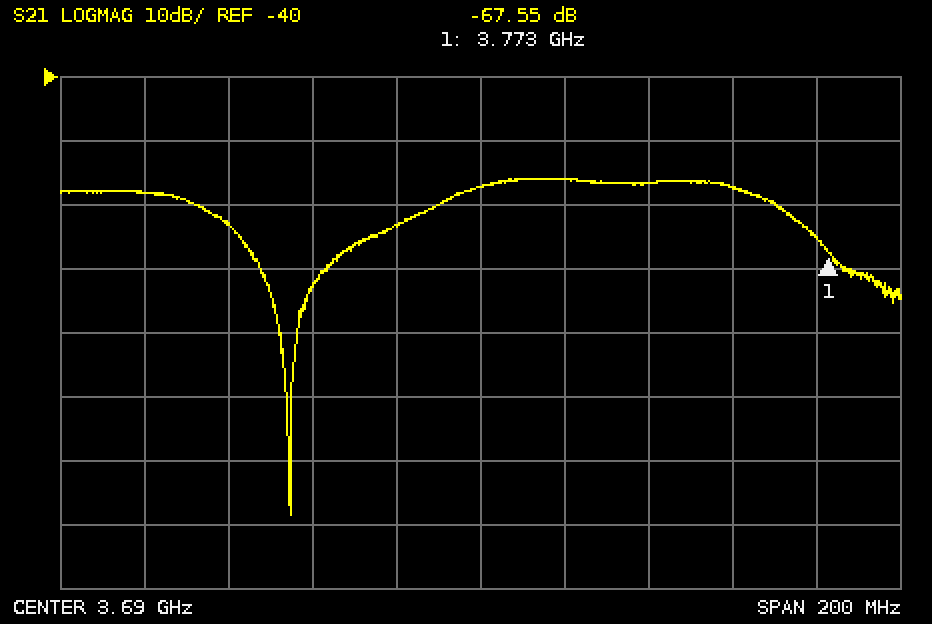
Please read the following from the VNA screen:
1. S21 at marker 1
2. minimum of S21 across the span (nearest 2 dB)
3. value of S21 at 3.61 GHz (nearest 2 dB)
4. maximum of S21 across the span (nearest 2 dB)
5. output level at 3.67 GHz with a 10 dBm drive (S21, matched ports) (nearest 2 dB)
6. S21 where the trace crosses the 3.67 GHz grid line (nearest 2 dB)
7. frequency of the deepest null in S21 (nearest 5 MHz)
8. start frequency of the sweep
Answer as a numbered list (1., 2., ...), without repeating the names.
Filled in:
1. -67.55 dB
2. -108 dB
3. -58 dB
4. -56 dB
5. -54 dBm
6. -64 dB
7. 3.645 GHz
8. 3.59 GHz
